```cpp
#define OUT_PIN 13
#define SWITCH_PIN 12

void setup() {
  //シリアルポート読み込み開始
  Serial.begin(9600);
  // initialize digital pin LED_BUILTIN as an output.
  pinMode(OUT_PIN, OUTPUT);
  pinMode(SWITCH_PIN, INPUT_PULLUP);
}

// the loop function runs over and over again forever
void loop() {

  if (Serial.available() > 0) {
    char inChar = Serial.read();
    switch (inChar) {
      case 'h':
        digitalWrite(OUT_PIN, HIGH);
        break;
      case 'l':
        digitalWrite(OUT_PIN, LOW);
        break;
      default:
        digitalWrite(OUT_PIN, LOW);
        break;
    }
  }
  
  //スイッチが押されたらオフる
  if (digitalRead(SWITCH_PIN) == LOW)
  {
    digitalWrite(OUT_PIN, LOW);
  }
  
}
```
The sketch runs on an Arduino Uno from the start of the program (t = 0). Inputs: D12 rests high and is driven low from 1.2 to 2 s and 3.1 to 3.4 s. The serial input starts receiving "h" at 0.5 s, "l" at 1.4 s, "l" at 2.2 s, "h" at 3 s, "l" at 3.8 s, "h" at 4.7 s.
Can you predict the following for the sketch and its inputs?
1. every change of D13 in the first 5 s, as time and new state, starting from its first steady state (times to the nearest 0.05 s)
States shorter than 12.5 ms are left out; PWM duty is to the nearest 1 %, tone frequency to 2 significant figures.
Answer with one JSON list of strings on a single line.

["0 s low; 0.5 s high; 1.2 s low; 3 s high; 3.1 s low; 4.7 s high"]
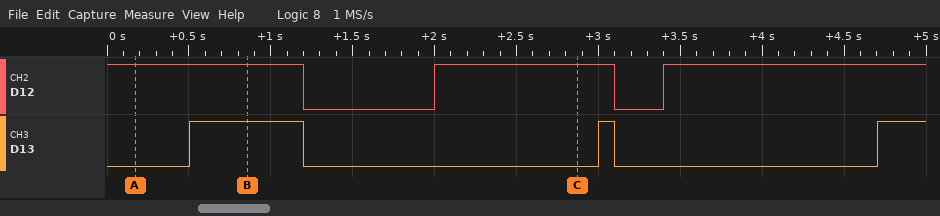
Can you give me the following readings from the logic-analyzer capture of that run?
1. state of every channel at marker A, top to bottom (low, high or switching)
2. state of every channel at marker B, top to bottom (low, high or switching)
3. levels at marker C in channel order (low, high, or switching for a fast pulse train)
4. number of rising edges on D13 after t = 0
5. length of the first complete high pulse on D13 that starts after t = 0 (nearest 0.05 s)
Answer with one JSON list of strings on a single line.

["D12 high, D13 low", "D12 high, D13 high", "D12 high, D13 low", "3", "0.70 s"]
